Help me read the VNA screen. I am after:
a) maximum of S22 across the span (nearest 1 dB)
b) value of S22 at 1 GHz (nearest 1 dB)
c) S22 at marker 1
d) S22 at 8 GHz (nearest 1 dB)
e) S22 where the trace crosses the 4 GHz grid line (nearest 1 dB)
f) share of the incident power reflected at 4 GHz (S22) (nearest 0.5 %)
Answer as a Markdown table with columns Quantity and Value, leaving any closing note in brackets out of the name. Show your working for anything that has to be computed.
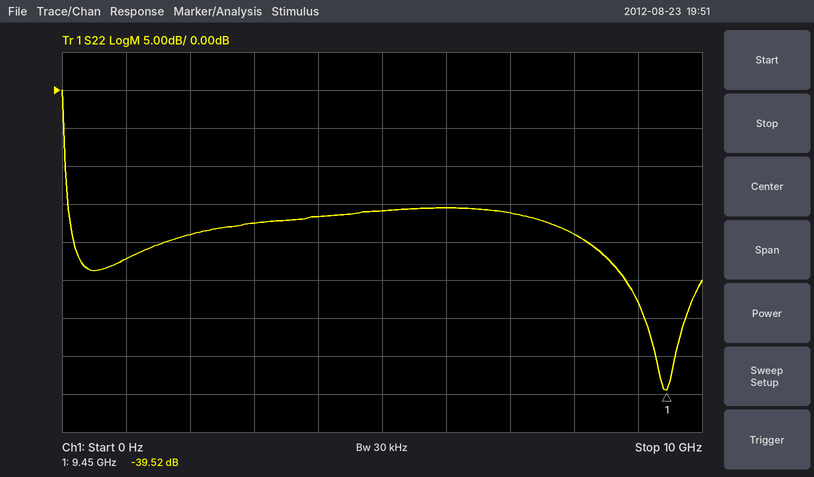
| Quantity | Value |
|---|---|
| maximum of S22 across the span | 0 dB |
| value of S22 at 1 GHz | -22 dB |
| S22 at marker 1 | -39.52 dB |
| S22 at 8 GHz | -19 dB |
| S22 where the trace crosses the 4 GHz grid line | -17 dB |
| share of the incident power reflected at 4 GHz (S22) | 10^(-17/10) ≈ 2.0 % |
